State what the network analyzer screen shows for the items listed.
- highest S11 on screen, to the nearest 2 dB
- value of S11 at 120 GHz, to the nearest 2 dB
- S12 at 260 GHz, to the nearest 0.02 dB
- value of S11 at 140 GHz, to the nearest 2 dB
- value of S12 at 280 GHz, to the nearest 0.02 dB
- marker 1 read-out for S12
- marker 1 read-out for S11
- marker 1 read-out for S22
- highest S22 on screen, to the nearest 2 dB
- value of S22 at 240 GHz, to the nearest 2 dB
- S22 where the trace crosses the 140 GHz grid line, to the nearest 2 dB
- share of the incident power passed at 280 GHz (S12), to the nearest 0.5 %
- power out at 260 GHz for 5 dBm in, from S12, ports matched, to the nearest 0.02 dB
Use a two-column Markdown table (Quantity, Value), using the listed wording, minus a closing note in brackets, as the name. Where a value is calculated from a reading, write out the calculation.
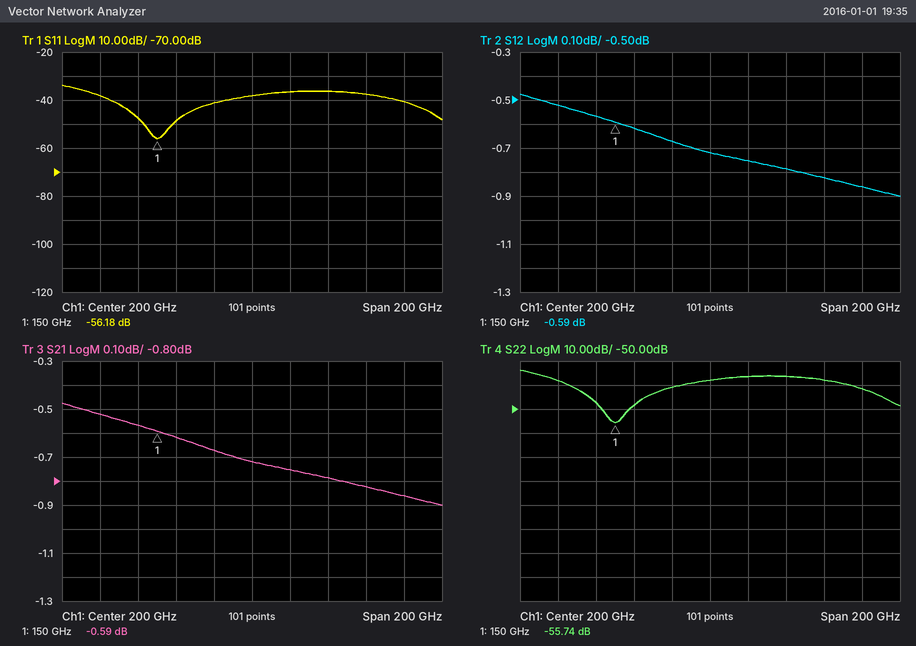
| Quantity | Value |
|---|---|
| highest S11 on screen, to the nearest 2 dB | -34 dB |
| value of S11 at 120 GHz, to the nearest 2 dB | -38 dB |
| S12 at 260 GHz, to the nearest 0.02 dB | -0.82 dB |
| value of S11 at 140 GHz, to the nearest 2 dB | -48 dB |
| value of S12 at 280 GHz, to the nearest 0.02 dB | -0.86 dB |
| marker 1 read-out for S12 | -0.59 dB |
| marker 1 read-out for S11 | -56.18 dB |
| marker 1 read-out for S22 | -55.74 dB |
| highest S22 on screen, to the nearest 2 dB | -34 dB |
| value of S22 at 240 GHz, to the nearest 2 dB | -36 dB |
| S22 where the trace crosses the 140 GHz grid line, to the nearest 2 dB | -48 dB |
| share of the incident power passed at 280 GHz (S12), to the nearest 0.5 % | 10^(-0.86/10) ≈ 82.0 % |
| power out at 260 GHz for 5 dBm in, from S12, ports matched, to the nearest 0.02 dB | 5 dBm + (-0.82 dB) = 4.18 dBm |
